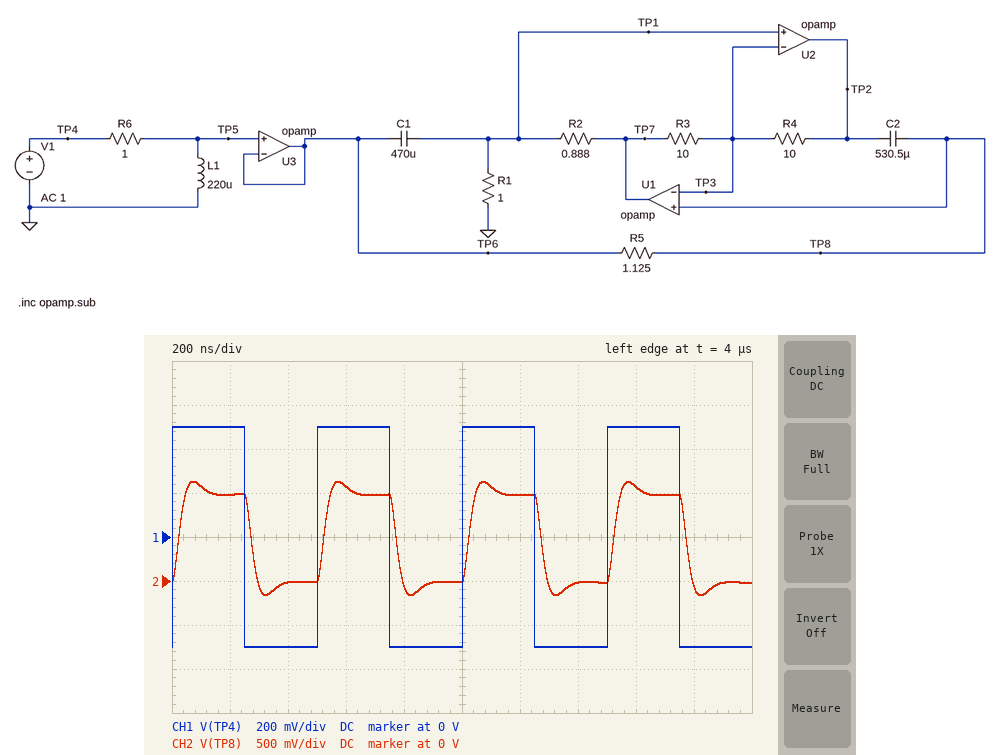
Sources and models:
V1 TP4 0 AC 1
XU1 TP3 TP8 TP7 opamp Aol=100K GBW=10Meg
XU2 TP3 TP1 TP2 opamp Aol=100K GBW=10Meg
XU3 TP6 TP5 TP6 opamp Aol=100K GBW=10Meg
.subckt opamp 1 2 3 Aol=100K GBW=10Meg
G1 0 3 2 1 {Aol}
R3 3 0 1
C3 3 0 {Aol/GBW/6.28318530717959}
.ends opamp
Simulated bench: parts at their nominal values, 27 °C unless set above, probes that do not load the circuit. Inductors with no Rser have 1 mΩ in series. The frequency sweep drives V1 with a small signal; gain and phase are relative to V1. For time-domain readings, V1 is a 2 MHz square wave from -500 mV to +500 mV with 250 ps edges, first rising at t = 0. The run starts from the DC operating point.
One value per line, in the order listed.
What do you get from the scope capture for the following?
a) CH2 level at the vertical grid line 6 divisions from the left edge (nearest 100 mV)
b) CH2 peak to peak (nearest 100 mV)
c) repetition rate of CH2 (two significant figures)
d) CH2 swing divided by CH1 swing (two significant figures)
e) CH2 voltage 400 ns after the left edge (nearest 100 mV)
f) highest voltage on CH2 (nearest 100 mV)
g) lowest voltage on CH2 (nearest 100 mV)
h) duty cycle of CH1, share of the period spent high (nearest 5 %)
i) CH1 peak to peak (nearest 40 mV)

1.0 V
1.3 V
2.0 MHz
1.3
0 V
1.1 V
-200 mV
50 %
1.00 V
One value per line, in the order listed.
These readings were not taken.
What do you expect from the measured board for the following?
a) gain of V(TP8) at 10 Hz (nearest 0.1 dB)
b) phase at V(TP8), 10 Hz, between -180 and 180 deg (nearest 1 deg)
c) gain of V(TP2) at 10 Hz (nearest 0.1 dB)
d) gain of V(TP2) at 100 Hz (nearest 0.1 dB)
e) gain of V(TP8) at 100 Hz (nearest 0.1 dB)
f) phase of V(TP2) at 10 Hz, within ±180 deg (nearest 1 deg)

-37.2 dB
83 deg
-56.3 dB
-54.2 dB
-17.8 dB
83 deg
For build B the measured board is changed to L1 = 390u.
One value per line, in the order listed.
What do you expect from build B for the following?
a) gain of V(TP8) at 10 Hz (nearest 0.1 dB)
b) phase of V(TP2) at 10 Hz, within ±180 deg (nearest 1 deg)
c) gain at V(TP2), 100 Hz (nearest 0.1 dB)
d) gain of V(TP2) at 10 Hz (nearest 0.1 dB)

-32.2 dB
84 deg
-49.4 dB
-51.3 dB
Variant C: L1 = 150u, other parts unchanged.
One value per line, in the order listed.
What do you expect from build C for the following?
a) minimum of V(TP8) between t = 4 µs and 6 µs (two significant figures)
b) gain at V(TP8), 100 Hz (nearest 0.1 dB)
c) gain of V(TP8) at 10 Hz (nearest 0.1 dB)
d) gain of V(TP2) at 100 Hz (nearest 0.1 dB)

-170 mV
-21.1 dB
-40.5 dB
-57.5 dB
